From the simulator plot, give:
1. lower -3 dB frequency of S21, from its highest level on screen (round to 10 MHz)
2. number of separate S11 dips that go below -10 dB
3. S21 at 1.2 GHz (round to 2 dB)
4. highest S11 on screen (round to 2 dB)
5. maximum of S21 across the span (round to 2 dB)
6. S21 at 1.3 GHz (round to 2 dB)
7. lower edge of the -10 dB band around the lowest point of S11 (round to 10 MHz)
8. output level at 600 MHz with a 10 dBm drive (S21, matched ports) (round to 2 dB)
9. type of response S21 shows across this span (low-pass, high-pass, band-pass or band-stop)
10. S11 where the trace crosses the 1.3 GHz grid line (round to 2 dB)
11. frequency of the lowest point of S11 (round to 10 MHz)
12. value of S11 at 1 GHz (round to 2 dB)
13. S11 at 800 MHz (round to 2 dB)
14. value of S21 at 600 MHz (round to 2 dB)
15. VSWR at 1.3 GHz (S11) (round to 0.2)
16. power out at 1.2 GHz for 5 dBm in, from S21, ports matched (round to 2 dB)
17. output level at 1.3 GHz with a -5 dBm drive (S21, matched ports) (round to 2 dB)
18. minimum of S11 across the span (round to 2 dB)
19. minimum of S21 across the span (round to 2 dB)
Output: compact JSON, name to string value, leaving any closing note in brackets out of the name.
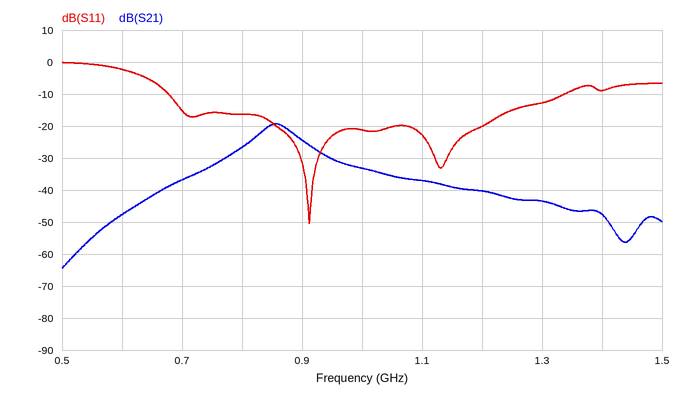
{"lower -3 dB frequency of S21, from its highest level on screen": "830 MHz", "number of separate S11 dips that go below -10 dB": "2", "S21 at 1.2 GHz": "-40 dB", "highest S11 on screen": "0 dB", "maximum of S21 across the span": "-20 dB", "S21 at 1.3 GHz": "-44 dB", "lower edge of the -10 dB band around the lowest point of S11": "680 MHz", "output level at 600 MHz with a 10 dBm drive (S21, matched ports)": "-38 dBm", "type of response S21 shows across this span": "band-pass", "S11 where the trace crosses the 1.3 GHz grid line": "-12 dB", "frequency of the lowest point of S11": "910 MHz", "value of S11 at 1 GHz": "-22 dB", "S11 at 800 MHz": "-16 dB", "value of S21 at 600 MHz": "-48 dB", "VSWR at 1.3 GHz (S11)": "1.6", "power out at 1.2 GHz for 5 dBm in, from S21, ports matched": "-36 dBm", "output level at 1.3 GHz with a -5 dBm drive (S21, matched ports)": "-48 dBm", "minimum of S11 across the span": "-50 dB", "minimum of S21 across the span": "-64 dB"}
